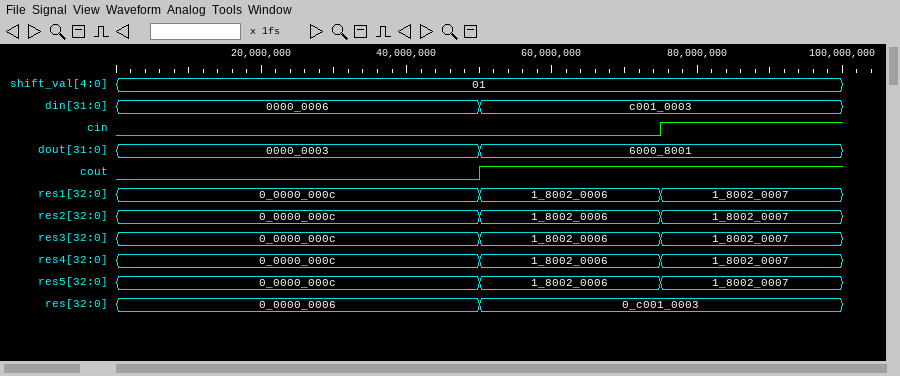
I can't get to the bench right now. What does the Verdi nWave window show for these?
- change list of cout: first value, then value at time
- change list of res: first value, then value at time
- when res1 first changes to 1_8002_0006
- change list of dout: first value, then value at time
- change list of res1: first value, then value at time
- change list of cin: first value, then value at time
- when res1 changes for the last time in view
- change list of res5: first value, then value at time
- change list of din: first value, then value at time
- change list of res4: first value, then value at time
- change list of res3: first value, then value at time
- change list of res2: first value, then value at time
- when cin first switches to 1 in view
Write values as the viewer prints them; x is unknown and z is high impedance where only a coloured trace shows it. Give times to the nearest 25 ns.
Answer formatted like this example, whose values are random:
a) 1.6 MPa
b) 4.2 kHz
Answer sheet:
a) 0, 1 at 50 ns
b) 0_0000_0006, 0_c001_0003 at 50 ns
c) 50 ns
d) 0000_0003, 6000_8001 at 50 ns
e) 0_0000_000c, 1_8002_0006 at 50 ns, 1_8002_0007 at 75 ns
f) 0, 1 at 75 ns
g) 75 ns
h) 0_0000_000c, 1_8002_0006 at 50 ns, 1_8002_0007 at 75 ns
i) 0000_0006, c001_0003 at 50 ns
j) 0_0000_000c, 1_8002_0006 at 50 ns, 1_8002_0007 at 75 ns
k) 0_0000_000c, 1_8002_0006 at 50 ns, 1_8002_0007 at 75 ns
l) 0_0000_000c, 1_8002_0006 at 50 ns, 1_8002_0007 at 75 ns
m) 75 ns
